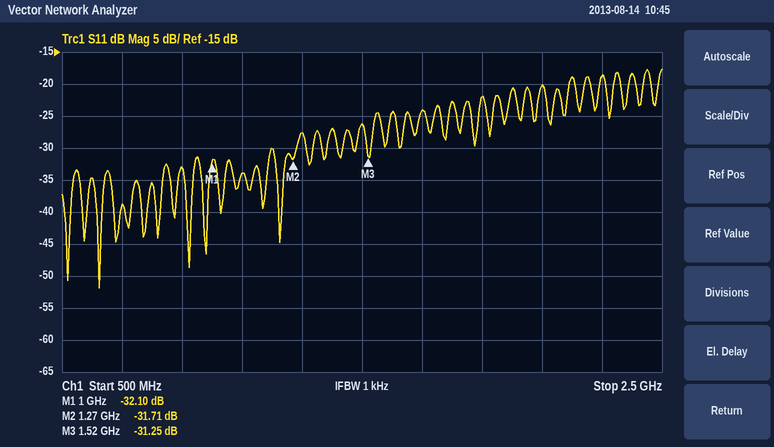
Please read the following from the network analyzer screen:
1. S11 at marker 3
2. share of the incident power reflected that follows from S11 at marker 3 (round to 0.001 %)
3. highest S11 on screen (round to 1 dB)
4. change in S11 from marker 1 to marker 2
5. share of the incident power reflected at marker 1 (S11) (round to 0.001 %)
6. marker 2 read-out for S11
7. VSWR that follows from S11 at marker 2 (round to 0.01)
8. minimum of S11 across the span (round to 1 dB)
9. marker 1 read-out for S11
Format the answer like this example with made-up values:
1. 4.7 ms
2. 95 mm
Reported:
1. -31.25 dB
2. 0.075 %
3. -18 dB
4. 0.39 dB
5. 0.062 %
6. -31.71 dB
7. 1.05
8. -52 dB
9. -32.10 dB
